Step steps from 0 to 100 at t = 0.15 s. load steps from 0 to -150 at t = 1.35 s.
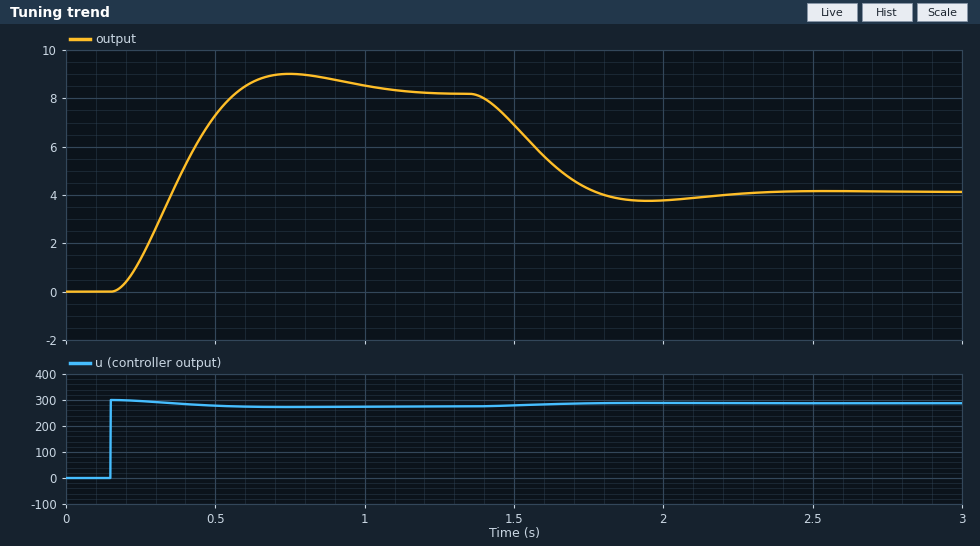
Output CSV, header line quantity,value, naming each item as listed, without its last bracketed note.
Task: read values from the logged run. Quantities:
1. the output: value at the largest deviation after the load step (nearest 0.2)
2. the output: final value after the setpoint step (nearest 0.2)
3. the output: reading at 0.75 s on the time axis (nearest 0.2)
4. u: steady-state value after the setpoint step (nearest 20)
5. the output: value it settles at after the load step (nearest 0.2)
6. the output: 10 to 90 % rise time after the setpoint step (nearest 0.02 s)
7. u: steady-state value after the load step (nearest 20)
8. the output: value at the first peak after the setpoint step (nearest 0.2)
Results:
quantity,value
the output: value at the largest deviation after the load step,3.8
the output: final value after the setpoint step,8.2
the output: reading at 0.75 s on the time axis,9.0
u: steady-state value after the setpoint step,280
the output: value it settles at after the load step,4.2
the output: 10 to 90 % rise time after the setpoint step,0.28 s
u: steady-state value after the load step,280
the output: value at the first peak after the setpoint step,9.0
